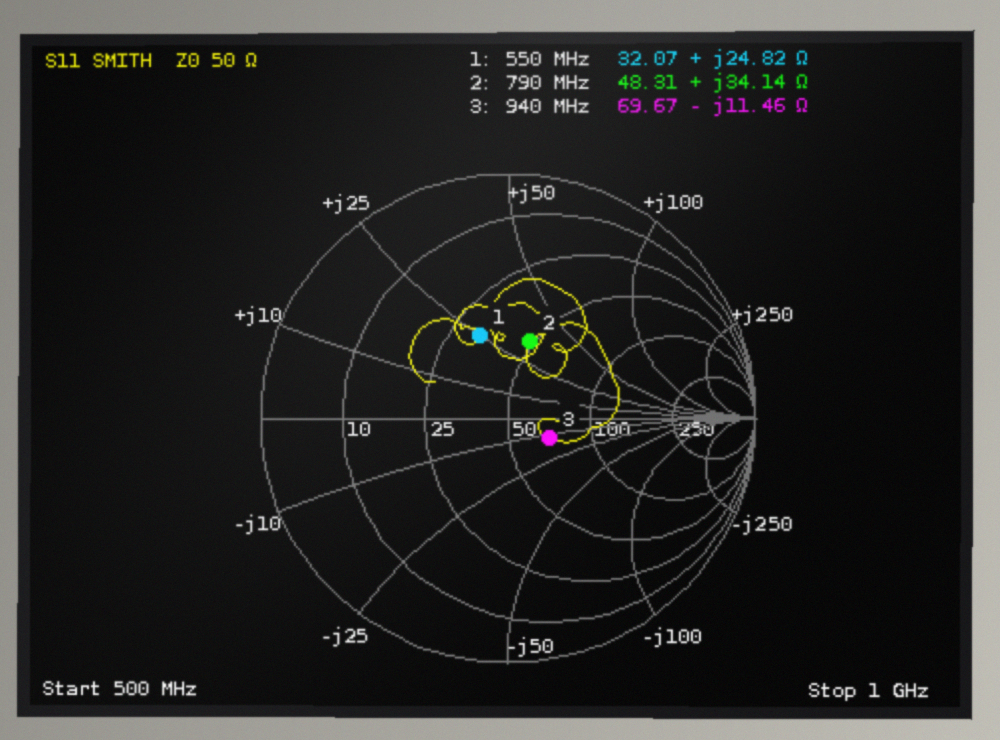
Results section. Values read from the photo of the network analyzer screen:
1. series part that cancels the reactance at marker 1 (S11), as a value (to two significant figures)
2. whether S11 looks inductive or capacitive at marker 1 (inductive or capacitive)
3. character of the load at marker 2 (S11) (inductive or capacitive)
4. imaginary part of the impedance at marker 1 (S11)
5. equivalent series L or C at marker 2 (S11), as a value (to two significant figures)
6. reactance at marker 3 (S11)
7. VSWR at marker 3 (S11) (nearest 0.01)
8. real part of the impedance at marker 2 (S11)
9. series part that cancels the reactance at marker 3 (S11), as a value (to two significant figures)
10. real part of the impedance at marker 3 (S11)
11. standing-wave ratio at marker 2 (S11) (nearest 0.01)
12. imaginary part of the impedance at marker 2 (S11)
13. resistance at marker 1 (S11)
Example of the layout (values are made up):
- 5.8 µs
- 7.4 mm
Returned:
- 12 pF
- inductive
- inductive
- +24.82 Ω
- 6.9 nH
- -11.46 Ω
- 1.47
- 48.31 Ω
- 1.9 nH
- 69.67 Ω
- 1.98
- +34.14 Ω
- 32.07 Ω
